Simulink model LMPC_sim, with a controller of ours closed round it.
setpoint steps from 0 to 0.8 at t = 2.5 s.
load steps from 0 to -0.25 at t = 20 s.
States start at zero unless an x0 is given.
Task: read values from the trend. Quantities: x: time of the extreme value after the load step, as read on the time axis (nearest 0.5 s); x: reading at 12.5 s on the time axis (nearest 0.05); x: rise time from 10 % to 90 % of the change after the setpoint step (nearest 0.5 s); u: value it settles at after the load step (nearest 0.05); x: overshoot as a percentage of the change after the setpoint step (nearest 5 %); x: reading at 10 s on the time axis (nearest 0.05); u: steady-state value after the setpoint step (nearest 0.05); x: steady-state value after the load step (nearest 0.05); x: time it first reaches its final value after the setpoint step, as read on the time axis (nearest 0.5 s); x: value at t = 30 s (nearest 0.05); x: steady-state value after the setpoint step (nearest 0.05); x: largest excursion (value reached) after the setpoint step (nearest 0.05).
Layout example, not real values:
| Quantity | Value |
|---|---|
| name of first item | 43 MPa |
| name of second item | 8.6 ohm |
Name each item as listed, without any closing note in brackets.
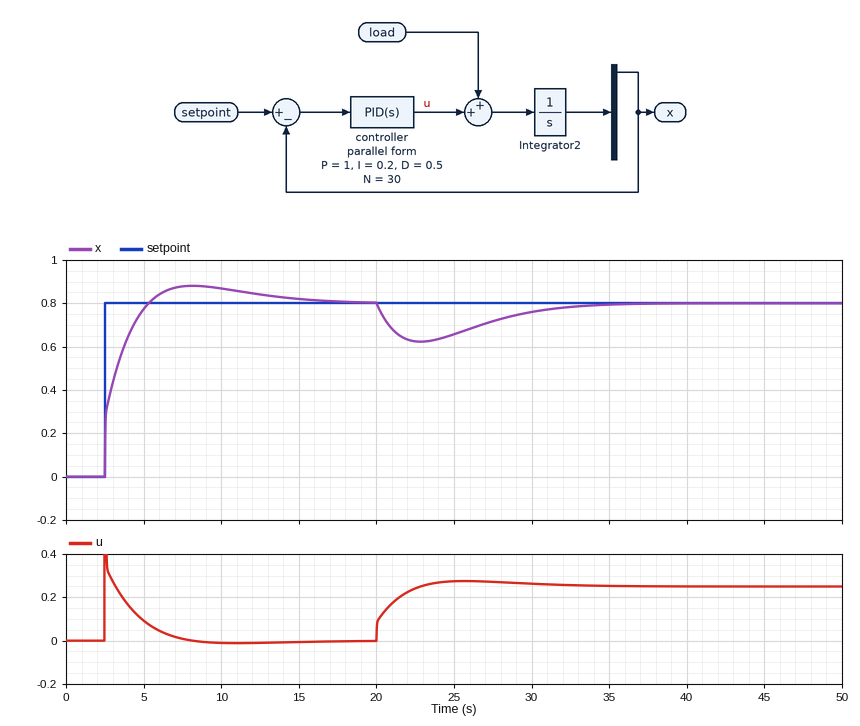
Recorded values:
| Quantity | Value |
|---|---|
| x: time of the extreme value after the load step, as read on the time axis | 23.0 s |
| x: reading at 12.5 s on the time axis | 0.85 |
| x: rise time from 10 % to 90 % of the change after the setpoint step | 2.0 s |
| u: value it settles at after the load step | 0.25 |
| x: overshoot as a percentage of the change after the setpoint step | 10 % |
| x: reading at 10 s on the time axis | 0.85 |
| u: steady-state value after the setpoint step | 0.00 |
| x: steady-state value after the load step | 0.80 |
| x: time it first reaches its final value after the setpoint step, as read on the time axis | 5.5 s |
| x: value at t = 30 s | 0.75 |
| x: steady-state value after the setpoint step | 0.80 |
| x: largest excursion (value reached) after the setpoint step | 0.90 |
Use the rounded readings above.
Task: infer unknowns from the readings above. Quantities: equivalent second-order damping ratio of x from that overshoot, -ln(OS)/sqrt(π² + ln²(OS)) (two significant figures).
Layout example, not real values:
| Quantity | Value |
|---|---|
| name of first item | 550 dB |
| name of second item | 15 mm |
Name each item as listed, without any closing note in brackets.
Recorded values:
| Quantity | Value |
|---|---|
| equivalent second-order damping ratio of x from that overshoot, -ln(OS)/sqrt(π² + ln²(OS)) | 0.59 |
